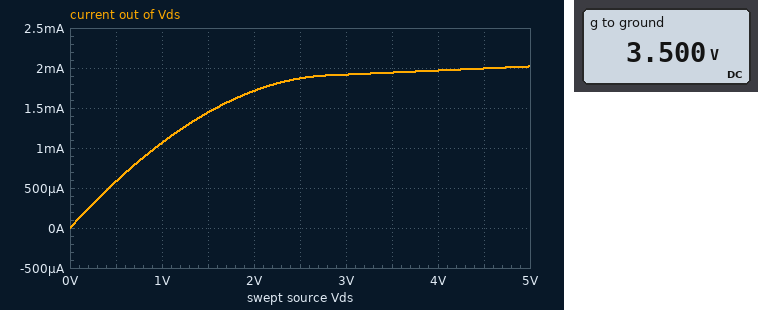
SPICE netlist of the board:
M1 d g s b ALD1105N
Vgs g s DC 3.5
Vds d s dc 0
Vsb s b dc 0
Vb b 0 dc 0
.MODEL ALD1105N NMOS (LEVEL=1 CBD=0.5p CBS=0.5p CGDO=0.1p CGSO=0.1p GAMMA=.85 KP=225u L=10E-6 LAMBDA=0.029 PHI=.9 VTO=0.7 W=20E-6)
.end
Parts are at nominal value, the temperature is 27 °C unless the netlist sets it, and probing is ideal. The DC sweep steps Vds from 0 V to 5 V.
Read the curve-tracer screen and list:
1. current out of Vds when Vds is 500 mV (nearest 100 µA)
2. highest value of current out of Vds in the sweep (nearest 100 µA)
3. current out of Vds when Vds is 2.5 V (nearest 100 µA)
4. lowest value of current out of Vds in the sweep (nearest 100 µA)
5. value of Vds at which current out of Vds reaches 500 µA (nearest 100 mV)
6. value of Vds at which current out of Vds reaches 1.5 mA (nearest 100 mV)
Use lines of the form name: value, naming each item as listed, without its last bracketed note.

current out of Vds when Vds is 500 mV: 600 µA
highest value of current out of Vds in the sweep: 2.0 mA
current out of Vds when Vds is 2.5 V: 1.9 mA
lowest value of current out of Vds in the sweep: 0 A
value of Vds at which current out of Vds reaches 500 µA: 400 mV
value of Vds at which current out of Vds reaches 1.5 mA: 1.6 V
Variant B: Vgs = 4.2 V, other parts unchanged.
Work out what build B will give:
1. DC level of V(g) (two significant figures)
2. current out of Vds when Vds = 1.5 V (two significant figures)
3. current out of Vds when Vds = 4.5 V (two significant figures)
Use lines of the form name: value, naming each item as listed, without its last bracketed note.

DC level of V(g): 4.2 V
current out of Vds when Vds = 1.5 V: 1.9 mA
current out of Vds when Vds = 4.5 V: 3.1 mA
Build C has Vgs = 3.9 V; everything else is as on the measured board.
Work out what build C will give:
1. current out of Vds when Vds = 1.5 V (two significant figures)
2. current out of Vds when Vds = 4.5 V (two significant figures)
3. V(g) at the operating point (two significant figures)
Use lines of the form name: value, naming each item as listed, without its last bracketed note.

current out of Vds when Vds = 1.5 V: 1.7 mA
current out of Vds when Vds = 4.5 V: 2.6 mA
V(g) at the operating point: 3.9 V
